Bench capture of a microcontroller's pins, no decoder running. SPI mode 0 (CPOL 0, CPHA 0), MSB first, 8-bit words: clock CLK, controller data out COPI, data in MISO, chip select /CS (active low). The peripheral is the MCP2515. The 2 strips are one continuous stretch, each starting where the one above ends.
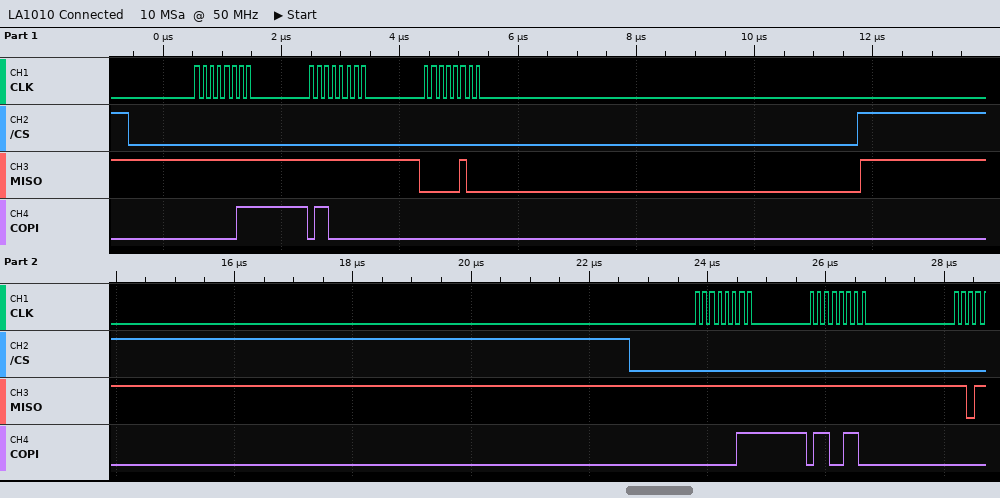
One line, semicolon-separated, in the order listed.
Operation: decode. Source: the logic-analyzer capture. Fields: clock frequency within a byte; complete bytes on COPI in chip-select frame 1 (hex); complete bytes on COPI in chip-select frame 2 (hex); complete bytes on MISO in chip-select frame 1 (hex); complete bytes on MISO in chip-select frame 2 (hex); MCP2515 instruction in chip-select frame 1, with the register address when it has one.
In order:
8 MHz; 03 60 00; 03 66; FF FF 04; FF FF; READ 0x60
